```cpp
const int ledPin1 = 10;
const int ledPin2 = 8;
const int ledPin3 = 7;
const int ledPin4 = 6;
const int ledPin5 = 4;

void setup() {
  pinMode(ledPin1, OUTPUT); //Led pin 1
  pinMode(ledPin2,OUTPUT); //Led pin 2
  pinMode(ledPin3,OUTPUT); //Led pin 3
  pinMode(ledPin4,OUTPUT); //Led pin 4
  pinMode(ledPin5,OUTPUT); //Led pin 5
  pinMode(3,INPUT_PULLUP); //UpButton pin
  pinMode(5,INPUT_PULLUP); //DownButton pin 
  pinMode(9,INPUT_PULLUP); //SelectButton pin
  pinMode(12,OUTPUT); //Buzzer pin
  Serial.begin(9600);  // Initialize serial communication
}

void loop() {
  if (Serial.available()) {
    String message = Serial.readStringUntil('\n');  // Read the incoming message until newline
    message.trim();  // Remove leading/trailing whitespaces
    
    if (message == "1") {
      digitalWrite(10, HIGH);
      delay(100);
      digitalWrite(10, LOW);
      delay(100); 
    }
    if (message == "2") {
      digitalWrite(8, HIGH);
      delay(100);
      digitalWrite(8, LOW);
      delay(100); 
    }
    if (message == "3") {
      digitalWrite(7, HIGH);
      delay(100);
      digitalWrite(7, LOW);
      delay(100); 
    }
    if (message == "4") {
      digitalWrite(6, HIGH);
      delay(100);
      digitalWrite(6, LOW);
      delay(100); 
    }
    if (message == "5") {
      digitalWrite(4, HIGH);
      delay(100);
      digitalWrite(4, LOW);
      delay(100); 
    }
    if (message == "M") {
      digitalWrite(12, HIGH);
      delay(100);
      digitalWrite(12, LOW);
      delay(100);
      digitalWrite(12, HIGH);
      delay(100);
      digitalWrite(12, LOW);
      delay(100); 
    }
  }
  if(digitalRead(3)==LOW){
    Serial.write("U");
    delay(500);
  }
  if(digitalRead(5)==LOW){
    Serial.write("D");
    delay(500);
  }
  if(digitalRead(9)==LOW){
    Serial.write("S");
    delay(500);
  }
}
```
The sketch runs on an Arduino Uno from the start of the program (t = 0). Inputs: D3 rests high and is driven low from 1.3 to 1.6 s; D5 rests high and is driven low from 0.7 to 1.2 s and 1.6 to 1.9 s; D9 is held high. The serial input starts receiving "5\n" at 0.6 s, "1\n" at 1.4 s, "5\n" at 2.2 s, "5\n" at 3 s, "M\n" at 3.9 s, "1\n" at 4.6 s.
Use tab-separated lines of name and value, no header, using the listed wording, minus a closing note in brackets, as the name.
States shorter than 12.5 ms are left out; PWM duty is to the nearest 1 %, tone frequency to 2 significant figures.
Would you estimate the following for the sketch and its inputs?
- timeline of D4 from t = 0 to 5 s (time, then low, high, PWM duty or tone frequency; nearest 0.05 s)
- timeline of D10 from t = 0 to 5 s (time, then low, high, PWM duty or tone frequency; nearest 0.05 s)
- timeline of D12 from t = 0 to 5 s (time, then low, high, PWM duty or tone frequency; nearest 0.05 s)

timeline of D4 from t = 0 to 5 s	0 s low; 0.6 s high; 0.7 s low; 2.5 s high; 2.6 s low; 3 s high; 3.1 s low
timeline of D10 from t = 0 to 5 s	0 s low; 2.3 s high; 2.4 s low; 4.6 s high; 4.7 s low
timeline of D12 from t = 0 to 5 s	0 s low; 3.9 s high; 4 s low; 4.1 s high; 4.2 s low
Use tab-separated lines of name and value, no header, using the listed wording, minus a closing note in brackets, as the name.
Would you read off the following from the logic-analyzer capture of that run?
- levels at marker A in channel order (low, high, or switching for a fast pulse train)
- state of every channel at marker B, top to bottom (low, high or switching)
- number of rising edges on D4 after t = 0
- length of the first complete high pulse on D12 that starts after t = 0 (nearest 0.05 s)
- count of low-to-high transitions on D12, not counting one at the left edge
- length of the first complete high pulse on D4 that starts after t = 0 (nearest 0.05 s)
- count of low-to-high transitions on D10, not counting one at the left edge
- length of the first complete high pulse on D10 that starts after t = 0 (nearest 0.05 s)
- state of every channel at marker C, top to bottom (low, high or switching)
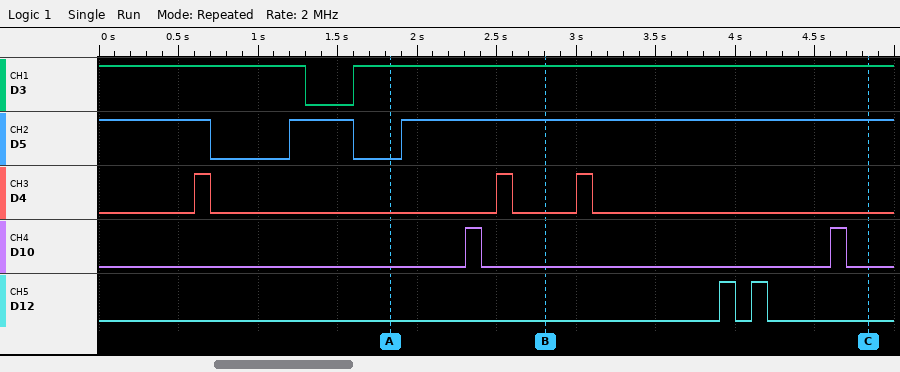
levels at marker A in channel order	D3 high, D5 low, D4 low, D10 low, D12 low
state of every channel at marker B, top to bottom	D3 high, D5 high, D4 low, D10 low, D12 low
number of rising edges on D4 after t = 0	3
length of the first complete high pulse on D12 that starts after t = 0	0.10 s
count of low-to-high transitions on D12, not counting one at the left edge	2
length of the first complete high pulse on D4 that starts after t = 0	0.10 s
count of low-to-high transitions on D10, not counting one at the left edge	2
length of the first complete high pulse on D10 that starts after t = 0	0.10 s
state of every channel at marker C, top to bottom	D3 high, D5 high, D4 low, D10 low, D12 low
